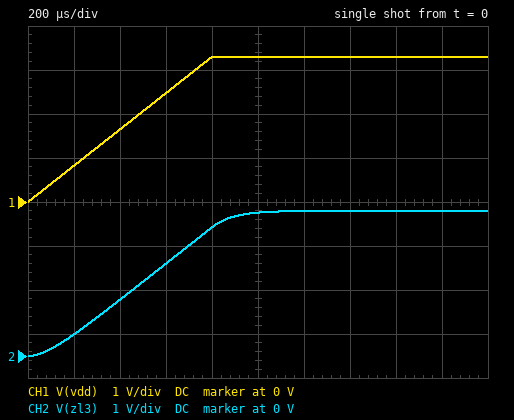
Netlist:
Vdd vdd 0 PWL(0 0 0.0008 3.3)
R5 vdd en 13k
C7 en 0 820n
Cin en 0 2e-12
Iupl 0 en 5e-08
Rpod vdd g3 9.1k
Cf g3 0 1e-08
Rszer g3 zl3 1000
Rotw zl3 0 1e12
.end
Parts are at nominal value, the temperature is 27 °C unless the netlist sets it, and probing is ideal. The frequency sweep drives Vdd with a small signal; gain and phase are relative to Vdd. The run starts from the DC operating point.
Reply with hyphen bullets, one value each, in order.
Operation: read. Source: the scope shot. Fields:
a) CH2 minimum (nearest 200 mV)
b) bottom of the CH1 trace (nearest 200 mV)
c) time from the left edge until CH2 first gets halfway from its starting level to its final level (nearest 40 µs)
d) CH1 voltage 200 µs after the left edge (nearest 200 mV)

- 0 V
- 0 V
- 480 µs
- 800 mV
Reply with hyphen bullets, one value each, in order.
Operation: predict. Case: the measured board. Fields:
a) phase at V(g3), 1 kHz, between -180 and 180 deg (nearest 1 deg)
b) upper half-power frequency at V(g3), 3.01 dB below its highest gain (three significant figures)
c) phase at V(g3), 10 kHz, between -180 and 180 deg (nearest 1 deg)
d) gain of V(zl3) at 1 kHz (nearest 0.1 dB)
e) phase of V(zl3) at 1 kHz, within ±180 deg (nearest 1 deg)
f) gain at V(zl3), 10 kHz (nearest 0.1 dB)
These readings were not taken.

- -30 deg
- 1.75 kHz
- -80 deg
- -1.2 dB
- -30 deg
- -15.3 dB
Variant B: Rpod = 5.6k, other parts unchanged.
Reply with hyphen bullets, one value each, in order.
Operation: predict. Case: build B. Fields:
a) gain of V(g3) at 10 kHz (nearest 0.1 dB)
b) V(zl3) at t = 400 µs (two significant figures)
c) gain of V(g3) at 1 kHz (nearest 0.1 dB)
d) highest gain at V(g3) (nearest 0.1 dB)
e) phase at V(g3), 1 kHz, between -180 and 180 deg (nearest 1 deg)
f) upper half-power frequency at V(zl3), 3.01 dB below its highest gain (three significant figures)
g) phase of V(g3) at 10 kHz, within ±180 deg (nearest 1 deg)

- -11.3 dB
- 1.4 V
- -0.5 dB
- 0 dB
- -19 deg
- 2.84 kHz
- -74 deg
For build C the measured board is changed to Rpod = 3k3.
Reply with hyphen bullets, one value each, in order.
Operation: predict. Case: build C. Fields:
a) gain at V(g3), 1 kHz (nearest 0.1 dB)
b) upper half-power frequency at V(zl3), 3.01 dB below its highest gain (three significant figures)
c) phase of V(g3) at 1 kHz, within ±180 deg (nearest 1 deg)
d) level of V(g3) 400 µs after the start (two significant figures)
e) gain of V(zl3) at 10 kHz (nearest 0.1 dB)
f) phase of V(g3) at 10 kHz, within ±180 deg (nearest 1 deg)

- -0.2 dB
- 4.82 kHz
- -12 deg
- 1.5 V
- -7.2 dB
- -64 deg
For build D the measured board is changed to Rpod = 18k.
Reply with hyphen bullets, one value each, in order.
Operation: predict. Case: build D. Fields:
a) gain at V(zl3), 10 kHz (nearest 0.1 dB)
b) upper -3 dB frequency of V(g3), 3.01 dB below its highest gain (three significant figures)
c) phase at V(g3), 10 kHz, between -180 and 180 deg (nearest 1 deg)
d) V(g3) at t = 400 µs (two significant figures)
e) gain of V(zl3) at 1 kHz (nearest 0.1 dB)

- -21.1 dB
- 884 Hz
- -85 deg
- 990 mV
- -3.6 dB
